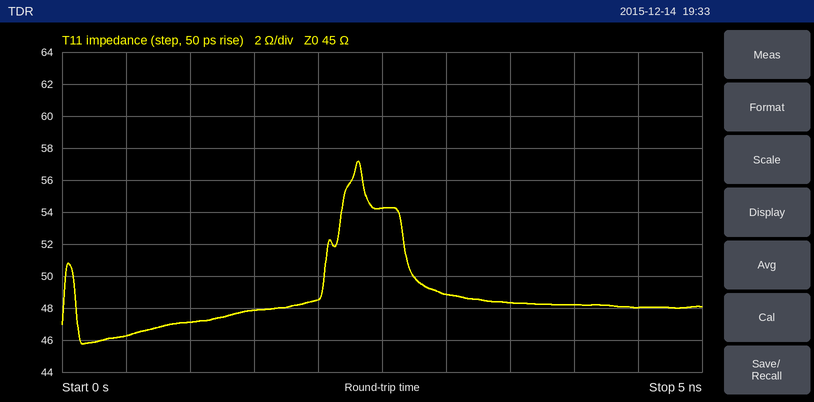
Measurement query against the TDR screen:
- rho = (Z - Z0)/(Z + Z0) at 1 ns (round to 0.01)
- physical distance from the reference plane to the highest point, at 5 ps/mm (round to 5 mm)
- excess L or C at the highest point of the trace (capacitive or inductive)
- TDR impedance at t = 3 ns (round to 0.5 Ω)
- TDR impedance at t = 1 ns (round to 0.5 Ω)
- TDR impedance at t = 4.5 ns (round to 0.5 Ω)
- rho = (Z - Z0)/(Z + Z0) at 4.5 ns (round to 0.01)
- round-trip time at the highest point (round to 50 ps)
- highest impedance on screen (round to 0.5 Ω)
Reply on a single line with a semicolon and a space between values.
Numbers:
+0.02; 230 mm; inductive; 49.0 Ω; 47.0 Ω; 48.0 Ω; +0.03; 2.30 ns; 57.0 Ω
